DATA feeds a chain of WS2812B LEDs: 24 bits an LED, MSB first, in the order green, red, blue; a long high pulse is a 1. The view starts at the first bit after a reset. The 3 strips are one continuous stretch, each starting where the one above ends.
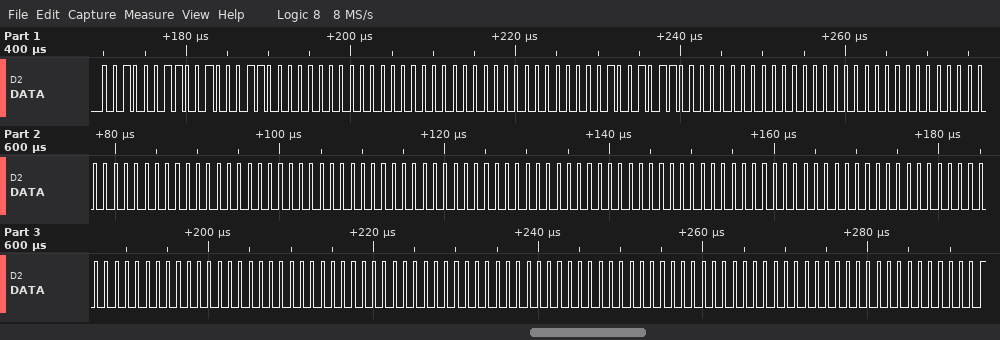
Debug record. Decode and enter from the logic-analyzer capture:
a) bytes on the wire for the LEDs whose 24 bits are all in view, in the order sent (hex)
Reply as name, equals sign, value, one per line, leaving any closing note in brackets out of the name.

bytes on the wire for the LEDs whose 24 bits are all in view, in the order sent = 23 23 00 00 00 00 4B 00 00 00 00 00 00 00 00 00 00 00 00 00 00 00 00 00 00 00 00 00 00 00
